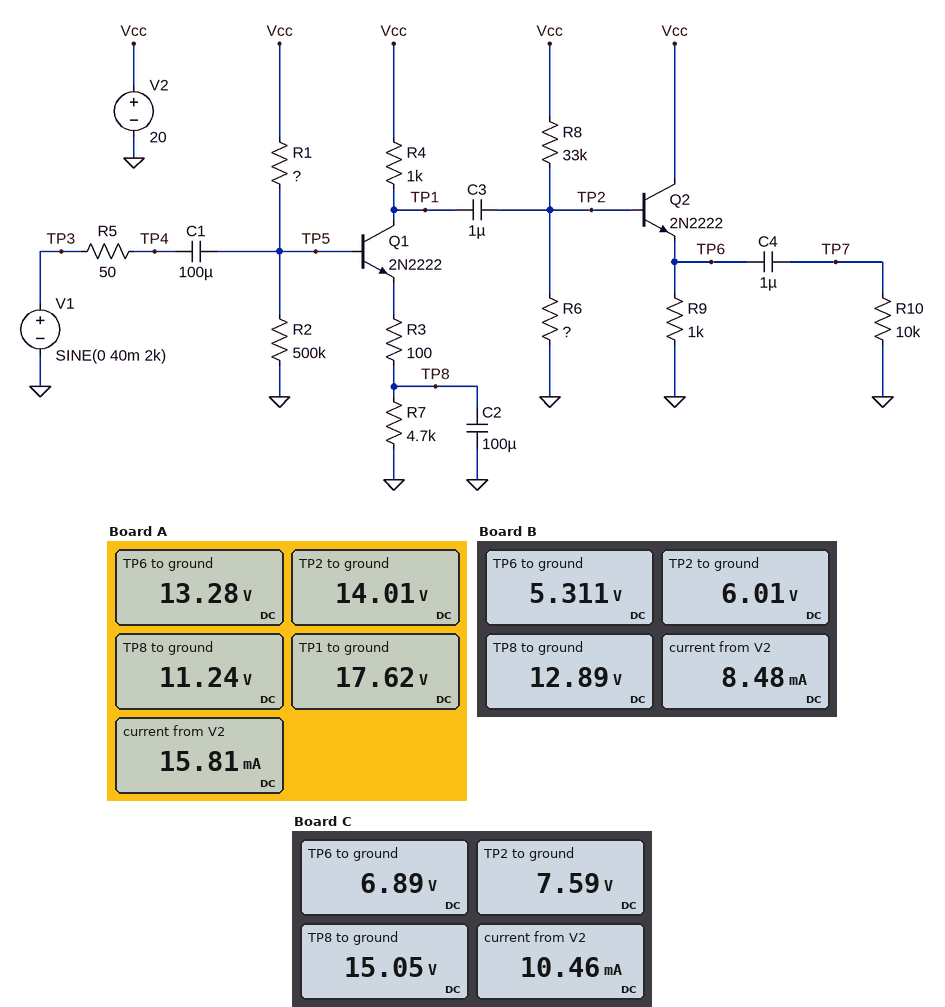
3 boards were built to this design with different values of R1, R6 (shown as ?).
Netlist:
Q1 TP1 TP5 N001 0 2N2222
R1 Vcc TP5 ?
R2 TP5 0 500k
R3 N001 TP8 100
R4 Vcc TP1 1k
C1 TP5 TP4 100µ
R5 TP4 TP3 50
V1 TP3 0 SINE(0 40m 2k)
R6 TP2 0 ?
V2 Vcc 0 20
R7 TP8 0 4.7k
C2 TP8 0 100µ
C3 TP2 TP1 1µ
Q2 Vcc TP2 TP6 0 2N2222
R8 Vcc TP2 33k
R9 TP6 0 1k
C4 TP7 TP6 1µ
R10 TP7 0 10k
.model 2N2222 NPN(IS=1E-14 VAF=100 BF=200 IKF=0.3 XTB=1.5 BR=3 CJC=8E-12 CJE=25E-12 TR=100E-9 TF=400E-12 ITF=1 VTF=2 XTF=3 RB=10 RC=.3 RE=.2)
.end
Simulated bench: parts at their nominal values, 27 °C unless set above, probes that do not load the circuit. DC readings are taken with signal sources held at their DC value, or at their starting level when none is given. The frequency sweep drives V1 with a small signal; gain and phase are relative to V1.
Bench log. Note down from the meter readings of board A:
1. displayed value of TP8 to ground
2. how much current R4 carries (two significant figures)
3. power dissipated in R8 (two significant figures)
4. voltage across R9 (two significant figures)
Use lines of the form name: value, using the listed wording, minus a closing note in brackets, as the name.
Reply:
displayed value of TP8 to ground: 11.24 V
how much current R4 carries: 2.4 mA
power dissipated in R8: 1.1 mW
voltage across R9: 13 V
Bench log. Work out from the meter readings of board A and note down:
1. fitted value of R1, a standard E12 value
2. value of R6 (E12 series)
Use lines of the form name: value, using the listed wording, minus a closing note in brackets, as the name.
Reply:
fitted value of R1, a standard E12 value: 220 kΩ
value of R6: 120 kΩ
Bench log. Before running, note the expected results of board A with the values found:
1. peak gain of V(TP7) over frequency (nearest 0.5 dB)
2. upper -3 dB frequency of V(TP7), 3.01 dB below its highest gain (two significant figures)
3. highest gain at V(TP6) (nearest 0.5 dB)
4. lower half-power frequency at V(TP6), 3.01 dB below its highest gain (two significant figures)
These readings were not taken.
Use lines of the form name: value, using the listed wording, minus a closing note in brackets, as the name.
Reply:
peak gain of V(TP7) over frequency: 18.5 dB
upper -3 dB frequency of V(TP7), 3.01 dB below its highest gain: 15 MHz
highest gain at V(TP6): 18.5 dB
lower half-power frequency at V(TP6), 3.01 dB below its highest gain: 17 Hz
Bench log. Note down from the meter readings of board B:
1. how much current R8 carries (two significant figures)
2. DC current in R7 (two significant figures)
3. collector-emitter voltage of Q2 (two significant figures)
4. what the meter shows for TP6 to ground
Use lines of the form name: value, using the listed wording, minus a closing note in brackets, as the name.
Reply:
how much current R8 carries: 420 µA
DC current in R7: 2.7 mA
collector-emitter voltage of Q2: 15 V
what the meter shows for TP6 to ground: 5.311 V
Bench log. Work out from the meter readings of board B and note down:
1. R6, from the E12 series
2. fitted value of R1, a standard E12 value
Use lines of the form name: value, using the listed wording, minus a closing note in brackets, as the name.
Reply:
R6, from the E12 series: 15 kΩ
fitted value of R1, a standard E12 value: 150 kΩ
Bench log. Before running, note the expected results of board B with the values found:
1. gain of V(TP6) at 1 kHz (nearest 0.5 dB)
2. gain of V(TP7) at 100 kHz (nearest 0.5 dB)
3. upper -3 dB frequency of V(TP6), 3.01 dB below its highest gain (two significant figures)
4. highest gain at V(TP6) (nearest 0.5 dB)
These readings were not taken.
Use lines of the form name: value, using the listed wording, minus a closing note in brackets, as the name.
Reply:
gain of V(TP6) at 1 kHz: 18.0 dB
gain of V(TP7) at 100 kHz: 18.0 dB
upper -3 dB frequency of V(TP6), 3.01 dB below its highest gain: 16 MHz
highest gain at V(TP6): 18.0 dB
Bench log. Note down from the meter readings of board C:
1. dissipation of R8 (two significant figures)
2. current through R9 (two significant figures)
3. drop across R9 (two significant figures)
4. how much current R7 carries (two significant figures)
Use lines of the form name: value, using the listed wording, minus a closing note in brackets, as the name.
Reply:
dissipation of R8: 4.7 mW
current through R9: 6.9 mA
drop across R9: 6.9 V
how much current R7 carries: 3.2 mA
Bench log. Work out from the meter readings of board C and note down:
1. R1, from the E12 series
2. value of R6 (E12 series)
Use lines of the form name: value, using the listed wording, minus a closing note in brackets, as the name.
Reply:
R1, from the E12 series: 82 kΩ
value of R6: 22 kΩ
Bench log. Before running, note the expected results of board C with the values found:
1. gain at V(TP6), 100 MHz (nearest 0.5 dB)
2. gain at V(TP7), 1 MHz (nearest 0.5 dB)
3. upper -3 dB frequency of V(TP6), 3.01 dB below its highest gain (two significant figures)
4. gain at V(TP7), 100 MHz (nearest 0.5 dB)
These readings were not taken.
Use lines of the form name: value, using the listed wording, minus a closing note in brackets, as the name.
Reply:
gain at V(TP6), 100 MHz: 1.0 dB
gain at V(TP7), 1 MHz: 18.5 dB
upper -3 dB frequency of V(TP6), 3.01 dB below its highest gain: 12 MHz
gain at V(TP7), 100 MHz: 1.0 dB
